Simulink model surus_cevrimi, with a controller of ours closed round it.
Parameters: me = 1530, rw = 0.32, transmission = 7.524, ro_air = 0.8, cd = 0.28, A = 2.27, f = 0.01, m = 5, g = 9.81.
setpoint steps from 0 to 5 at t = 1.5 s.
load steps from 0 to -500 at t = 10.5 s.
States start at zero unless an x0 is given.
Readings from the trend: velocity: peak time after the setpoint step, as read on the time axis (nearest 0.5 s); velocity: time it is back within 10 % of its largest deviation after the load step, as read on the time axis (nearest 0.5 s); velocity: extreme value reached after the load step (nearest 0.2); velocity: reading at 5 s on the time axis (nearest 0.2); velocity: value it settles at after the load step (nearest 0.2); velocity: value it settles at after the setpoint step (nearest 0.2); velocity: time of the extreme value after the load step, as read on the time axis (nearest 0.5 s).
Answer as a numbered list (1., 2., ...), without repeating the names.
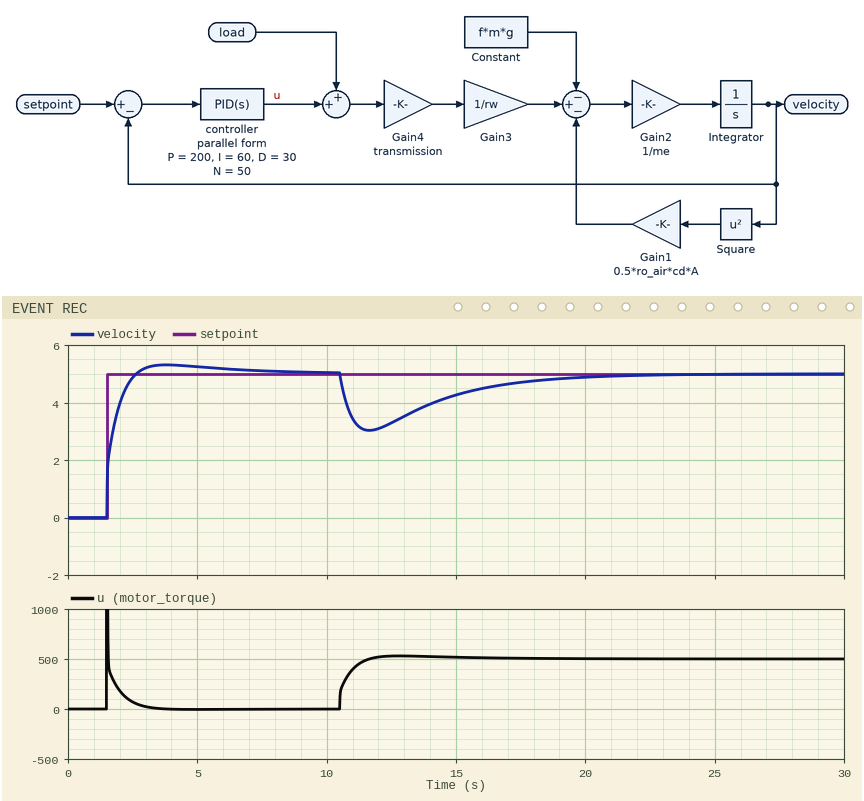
1. 4.0 s
2. 18.5 s
3. 3.0
4. 5.2
5. 5.0
6. 5.0
7. 11.5 s
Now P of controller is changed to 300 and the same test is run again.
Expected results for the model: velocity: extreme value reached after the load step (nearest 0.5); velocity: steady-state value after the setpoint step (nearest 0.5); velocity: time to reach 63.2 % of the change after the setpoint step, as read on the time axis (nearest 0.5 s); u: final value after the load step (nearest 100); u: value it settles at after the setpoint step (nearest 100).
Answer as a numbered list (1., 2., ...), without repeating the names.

1. 3.5
2. 5.0
3. 1.5 s
4. 500
5. 0
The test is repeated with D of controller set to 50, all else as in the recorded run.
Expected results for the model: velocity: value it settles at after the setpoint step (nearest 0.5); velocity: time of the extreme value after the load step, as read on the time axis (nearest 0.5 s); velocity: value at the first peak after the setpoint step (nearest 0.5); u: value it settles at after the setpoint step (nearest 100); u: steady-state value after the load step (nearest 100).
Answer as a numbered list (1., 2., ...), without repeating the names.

1. 5.0
2. 12.0 s
3. 5.5
4. 0
5. 500
